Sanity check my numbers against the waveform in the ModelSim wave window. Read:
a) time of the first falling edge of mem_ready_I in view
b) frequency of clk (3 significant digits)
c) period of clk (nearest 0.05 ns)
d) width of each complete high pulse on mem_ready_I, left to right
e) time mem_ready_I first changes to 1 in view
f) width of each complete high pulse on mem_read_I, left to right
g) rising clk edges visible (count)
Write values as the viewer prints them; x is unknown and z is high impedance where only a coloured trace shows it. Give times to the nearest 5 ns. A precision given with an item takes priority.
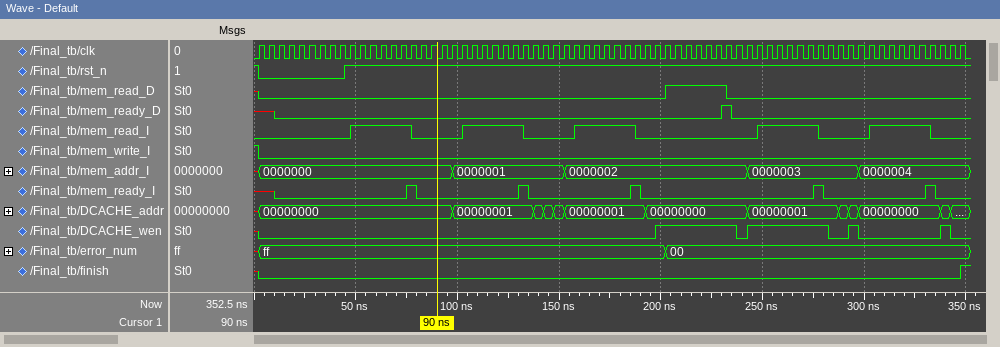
80 ns
200 MHz
5 ns
5 ns, 5 ns, 5 ns, 5 ns, 5 ns
75 ns
30 ns, 30 ns, 30 ns, 30 ns, 30 ns
70
